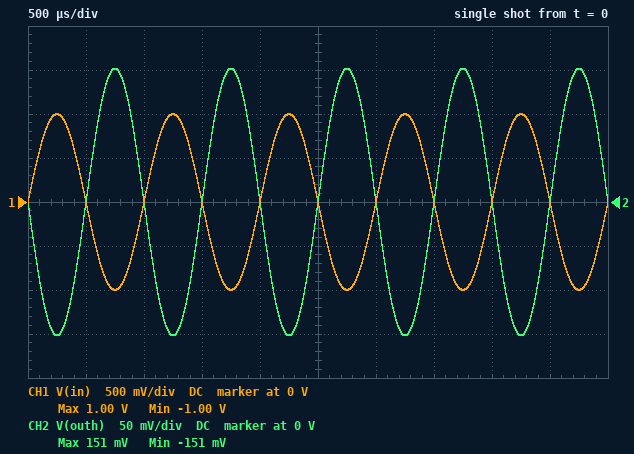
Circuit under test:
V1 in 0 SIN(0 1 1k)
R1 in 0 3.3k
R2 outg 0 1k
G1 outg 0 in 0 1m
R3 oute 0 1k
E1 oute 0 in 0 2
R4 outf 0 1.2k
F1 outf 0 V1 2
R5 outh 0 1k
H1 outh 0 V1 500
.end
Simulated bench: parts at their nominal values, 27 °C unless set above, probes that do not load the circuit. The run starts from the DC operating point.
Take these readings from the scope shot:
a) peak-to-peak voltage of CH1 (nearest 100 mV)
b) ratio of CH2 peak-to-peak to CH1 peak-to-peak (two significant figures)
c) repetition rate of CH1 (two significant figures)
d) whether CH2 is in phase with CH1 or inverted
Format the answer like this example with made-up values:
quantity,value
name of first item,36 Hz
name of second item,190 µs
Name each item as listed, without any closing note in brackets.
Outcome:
quantity,value
peak-to-peak voltage of CH1,2.0 V
ratio of CH2 peak-to-peak to CH1 peak-to-peak,0.15
repetition rate of CH1,1.0 kHz
whether CH2 is in phase with CH1 or inverted,inverted
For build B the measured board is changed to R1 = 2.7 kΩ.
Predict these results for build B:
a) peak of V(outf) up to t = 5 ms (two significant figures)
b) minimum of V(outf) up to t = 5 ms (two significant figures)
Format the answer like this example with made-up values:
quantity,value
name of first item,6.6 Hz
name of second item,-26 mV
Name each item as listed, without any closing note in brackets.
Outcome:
quantity,value
peak of V(outf) up to t = 5 ms,890 mV
minimum of V(outf) up to t = 5 ms,-890 mV
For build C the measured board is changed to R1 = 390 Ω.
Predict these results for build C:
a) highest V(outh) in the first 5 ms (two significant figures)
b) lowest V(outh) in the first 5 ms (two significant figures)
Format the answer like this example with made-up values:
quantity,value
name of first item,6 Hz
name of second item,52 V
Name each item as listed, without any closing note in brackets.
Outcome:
quantity,value
highest V(outh) in the first 5 ms,1.3 V
lowest V(outh) in the first 5 ms,-1.3 V
